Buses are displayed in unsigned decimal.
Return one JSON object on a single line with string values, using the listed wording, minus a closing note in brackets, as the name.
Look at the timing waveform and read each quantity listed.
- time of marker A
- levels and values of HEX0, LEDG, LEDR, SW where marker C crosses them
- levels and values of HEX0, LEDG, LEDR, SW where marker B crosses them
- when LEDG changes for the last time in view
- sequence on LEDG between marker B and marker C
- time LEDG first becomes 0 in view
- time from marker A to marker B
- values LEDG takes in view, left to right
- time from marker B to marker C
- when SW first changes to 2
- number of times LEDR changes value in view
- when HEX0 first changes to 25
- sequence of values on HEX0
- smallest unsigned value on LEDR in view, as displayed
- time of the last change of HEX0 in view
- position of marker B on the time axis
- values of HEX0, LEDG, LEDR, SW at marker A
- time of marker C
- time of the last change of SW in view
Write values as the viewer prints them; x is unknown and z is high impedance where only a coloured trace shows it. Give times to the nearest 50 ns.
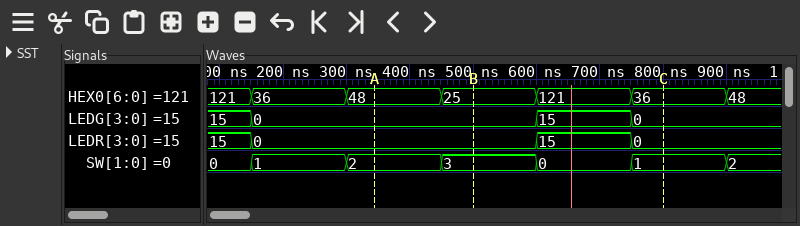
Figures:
{"time of marker A": "350 ns", "levels and values of HEX0, LEDG, LEDR, SW where marker C crosses them": "HEX0=36, LEDG=0, LEDR=0, SW=1", "levels and values of HEX0, LEDG, LEDR, SW where marker B crosses them": "HEX0=25, LEDG=0, LEDR=0, SW=3", "when LEDG changes for the last time in view": "750 ns", "sequence on LEDG between marker B and marker C": "0, 15, 0", "time LEDG first becomes 0 in view": "150 ns", "time from marker A to marker B": "150 ns", "values LEDG takes in view, left to right": "15, 0, 15, 0", "time from marker B to marker C": "300 ns", "when SW first changes to 2": "300 ns", "number of times LEDR changes value in view": "3", "when HEX0 first changes to 25": "450 ns", "sequence of values on HEX0": "121, 36, 48, 25, 121, 36, 48", "smallest unsigned value on LEDR in view, as displayed": "0", "time of the last change of HEX0 in view": "900 ns", "position of marker B on the time axis": "500 ns", "values of HEX0, LEDG, LEDR, SW at marker A": "HEX0=48, LEDG=0, LEDR=0, SW=2", "time of marker C": "800 ns", "time of the last change of SW in view": "900 ns"}
